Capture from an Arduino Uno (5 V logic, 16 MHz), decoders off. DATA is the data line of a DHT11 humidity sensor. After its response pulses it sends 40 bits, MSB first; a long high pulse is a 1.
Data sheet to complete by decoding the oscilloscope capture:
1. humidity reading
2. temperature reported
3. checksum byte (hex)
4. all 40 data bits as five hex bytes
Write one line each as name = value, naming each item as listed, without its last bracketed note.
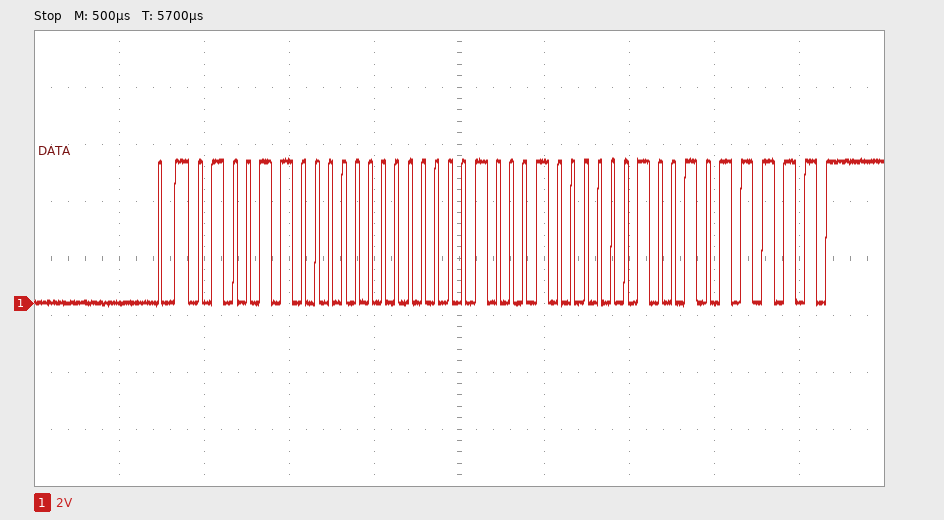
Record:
humidity reading = 76 %
temperature reported = 17.2 °C
checksum byte = 0x5F
all 40 data bits as five hex bytes = 4C 00 11 02 5F
